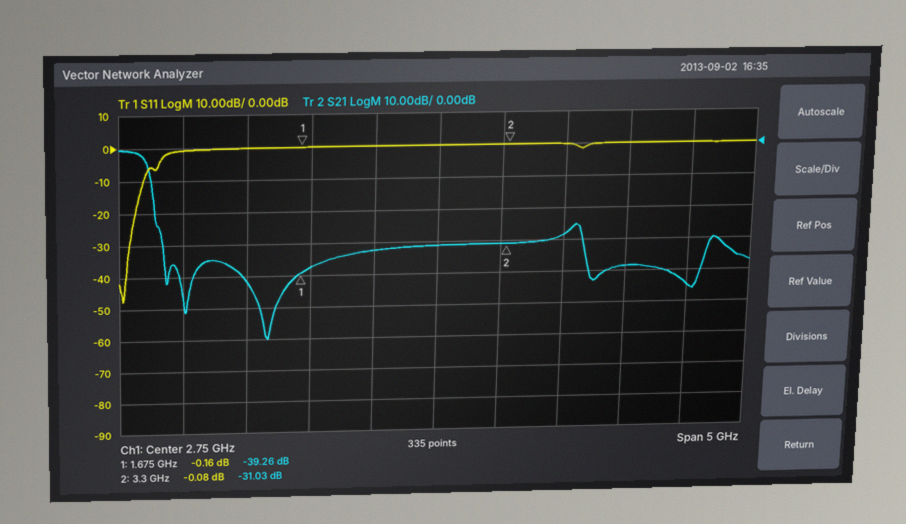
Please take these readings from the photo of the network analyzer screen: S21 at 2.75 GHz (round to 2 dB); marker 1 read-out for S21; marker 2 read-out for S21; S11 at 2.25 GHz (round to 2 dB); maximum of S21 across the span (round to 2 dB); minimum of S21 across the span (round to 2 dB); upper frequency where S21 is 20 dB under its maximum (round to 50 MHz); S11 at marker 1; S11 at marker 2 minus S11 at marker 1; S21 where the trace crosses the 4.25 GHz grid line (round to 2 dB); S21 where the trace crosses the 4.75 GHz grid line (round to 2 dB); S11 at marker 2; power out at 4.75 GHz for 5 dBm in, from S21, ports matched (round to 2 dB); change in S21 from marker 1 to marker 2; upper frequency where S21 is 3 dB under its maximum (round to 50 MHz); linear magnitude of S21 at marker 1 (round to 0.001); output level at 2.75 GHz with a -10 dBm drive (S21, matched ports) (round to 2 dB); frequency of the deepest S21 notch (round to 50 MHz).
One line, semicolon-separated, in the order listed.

-32 dB; -39.26 dB; -31.03 dB; 0 dB; 0 dB; -60 dB; 550 MHz; -0.16 dB; 0.08 dB; -38 dB; -44 dB; -0.08 dB; -40 dBm; 8.23 dB; 450 MHz; 0.011; -42 dBm; 1.40 GHz
